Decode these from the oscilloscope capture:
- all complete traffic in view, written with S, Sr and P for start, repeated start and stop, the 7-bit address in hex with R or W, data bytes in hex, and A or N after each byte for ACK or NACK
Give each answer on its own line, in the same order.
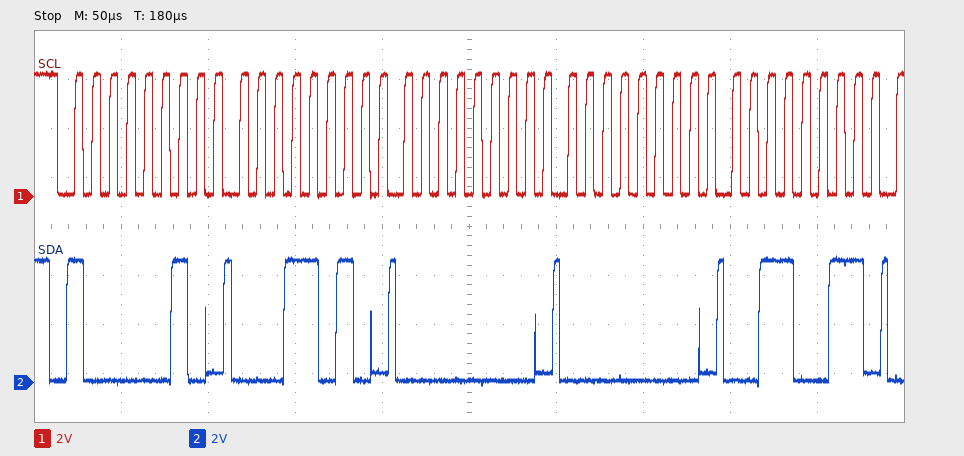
S 41W A 1A A 00 A 00 A 33 A
